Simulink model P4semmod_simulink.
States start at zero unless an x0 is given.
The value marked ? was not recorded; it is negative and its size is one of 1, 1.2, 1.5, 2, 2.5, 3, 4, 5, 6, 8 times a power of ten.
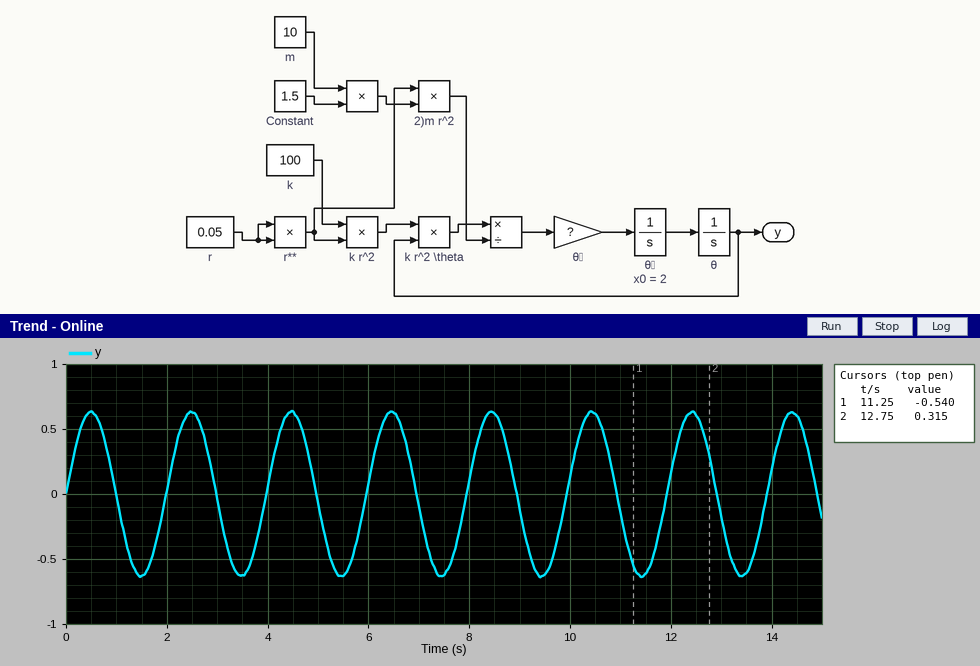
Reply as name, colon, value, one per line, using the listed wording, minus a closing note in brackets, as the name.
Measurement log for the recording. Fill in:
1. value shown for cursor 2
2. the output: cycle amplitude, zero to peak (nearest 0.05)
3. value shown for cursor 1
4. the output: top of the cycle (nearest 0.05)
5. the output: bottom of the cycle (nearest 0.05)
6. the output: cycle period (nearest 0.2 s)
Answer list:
value shown for cursor 2: 0.315
the output: cycle amplitude, zero to peak: 0.65
value shown for cursor 1: -0.540
the output: top of the cycle: 0.65
the output: bottom of the cycle: -0.65
the output: cycle period: 2.0 s
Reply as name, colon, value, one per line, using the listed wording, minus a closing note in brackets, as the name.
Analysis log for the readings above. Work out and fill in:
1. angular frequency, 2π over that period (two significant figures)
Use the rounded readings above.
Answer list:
angular frequency, 2π over that period: 3.1 rad/s
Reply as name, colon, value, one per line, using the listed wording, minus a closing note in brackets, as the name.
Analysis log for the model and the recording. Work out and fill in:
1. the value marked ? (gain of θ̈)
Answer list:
the value marked ?: -1.5
